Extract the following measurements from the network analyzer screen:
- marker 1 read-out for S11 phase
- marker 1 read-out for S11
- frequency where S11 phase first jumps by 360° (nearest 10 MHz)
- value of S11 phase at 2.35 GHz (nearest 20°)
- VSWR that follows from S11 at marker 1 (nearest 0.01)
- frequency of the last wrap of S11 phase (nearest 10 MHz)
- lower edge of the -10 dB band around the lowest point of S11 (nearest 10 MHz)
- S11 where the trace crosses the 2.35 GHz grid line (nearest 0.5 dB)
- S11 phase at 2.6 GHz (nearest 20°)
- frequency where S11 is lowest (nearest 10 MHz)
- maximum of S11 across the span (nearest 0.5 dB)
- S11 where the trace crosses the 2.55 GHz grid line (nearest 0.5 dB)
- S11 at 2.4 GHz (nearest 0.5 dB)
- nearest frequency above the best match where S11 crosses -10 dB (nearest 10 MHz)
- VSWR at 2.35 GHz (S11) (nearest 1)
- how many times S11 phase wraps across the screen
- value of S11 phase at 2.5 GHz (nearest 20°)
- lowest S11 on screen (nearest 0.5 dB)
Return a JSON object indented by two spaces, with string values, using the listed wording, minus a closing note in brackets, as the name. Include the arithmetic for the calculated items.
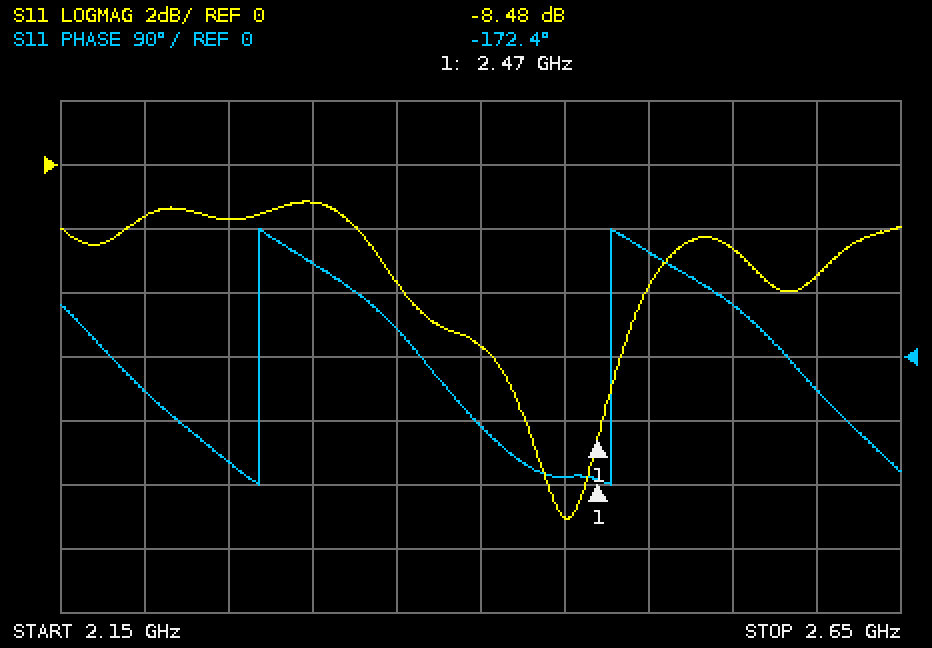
{
  "marker 1 read-out for S11 phase": "-172.4°",
  "marker 1 read-out for S11": "-8.48 dB",
  "frequency where S11 phase first jumps by 360°": "2.27 GHz",
  "value of S11 phase at 2.35 GHz": "40°",
  "VSWR that follows from S11 at marker 1": "(1 + 0.3767)/(1 − 0.3767) ≈ 2.21",
  "frequency of the last wrap of S11 phase": "2.48 GHz",
  "lower edge of the -10 dB band around the lowest point of S11": "2.44 GHz",
  "S11 where the trace crosses the 2.35 GHz grid line": "-3.5 dB",
  "S11 phase at 2.6 GHz": "-40°",
  "frequency where S11 is lowest": "2.45 GHz",
  "maximum of S11 across the span": "-1.0 dB",
  "S11 where the trace crosses the 2.55 GHz grid line": "-2.5 dB",
  "S11 at 2.4 GHz": "-5.5 dB",
  "nearest frequency above the best match where S11 crosses -10 dB": "2.46 GHz",
  "VSWR at 2.35 GHz (S11)": "|Γ| = 10^(-3.5/20) = 0.6683; VSWR = (1 + 0.6683)/(1 − 0.6683) ≈ 5",
  "how many times S11 phase wraps across the screen": "2",
  "value of S11 phase at 2.5 GHz": "140°",
  "lowest S11 on screen": "-11.0 dB"
}
